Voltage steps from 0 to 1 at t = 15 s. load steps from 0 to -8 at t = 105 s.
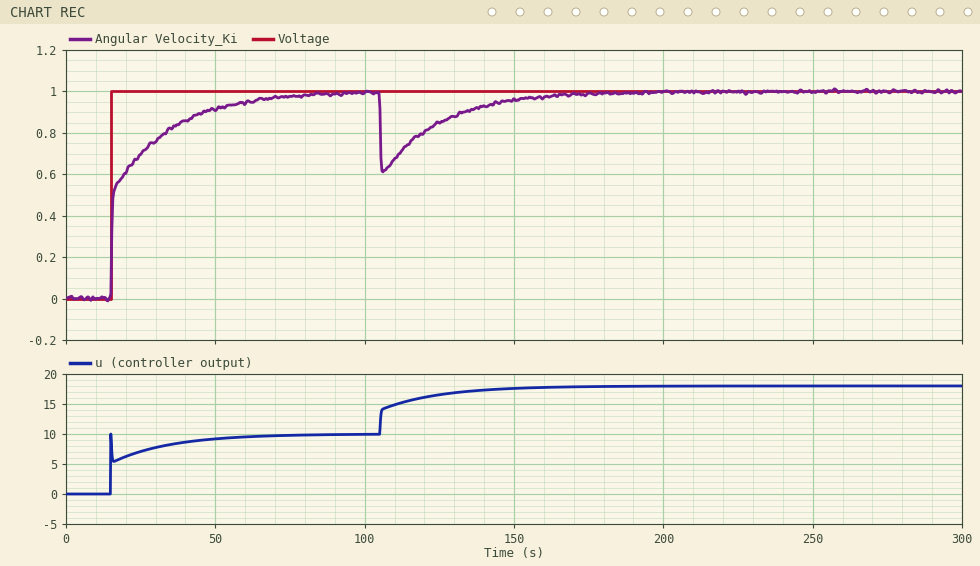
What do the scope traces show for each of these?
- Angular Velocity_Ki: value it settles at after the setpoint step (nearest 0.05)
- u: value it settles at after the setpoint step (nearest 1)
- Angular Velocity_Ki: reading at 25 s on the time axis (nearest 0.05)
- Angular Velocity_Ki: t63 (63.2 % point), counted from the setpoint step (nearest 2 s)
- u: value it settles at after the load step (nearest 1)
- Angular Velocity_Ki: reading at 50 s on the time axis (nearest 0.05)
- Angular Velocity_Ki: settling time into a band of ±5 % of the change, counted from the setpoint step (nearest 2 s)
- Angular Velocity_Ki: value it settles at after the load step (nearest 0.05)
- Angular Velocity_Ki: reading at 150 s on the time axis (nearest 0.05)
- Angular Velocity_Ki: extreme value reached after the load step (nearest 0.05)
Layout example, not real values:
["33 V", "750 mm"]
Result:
["1.00", "10", "0.70", "6 s", "18", "0.90", "46 s", "1.00", "0.95", "0.60"]
